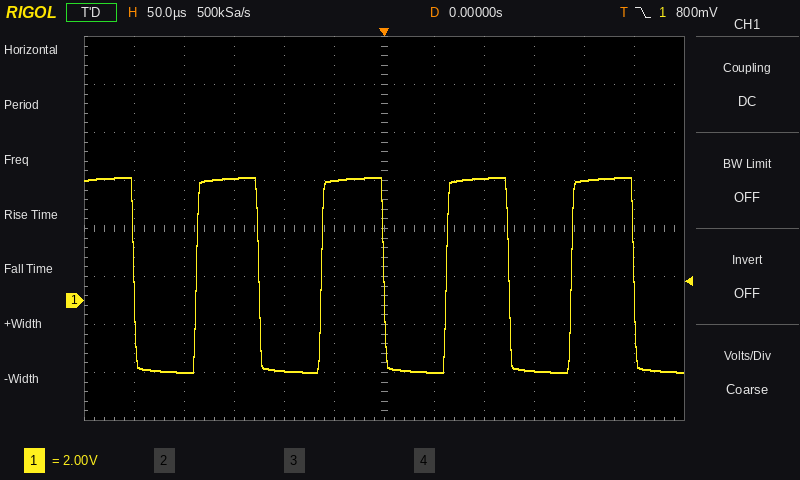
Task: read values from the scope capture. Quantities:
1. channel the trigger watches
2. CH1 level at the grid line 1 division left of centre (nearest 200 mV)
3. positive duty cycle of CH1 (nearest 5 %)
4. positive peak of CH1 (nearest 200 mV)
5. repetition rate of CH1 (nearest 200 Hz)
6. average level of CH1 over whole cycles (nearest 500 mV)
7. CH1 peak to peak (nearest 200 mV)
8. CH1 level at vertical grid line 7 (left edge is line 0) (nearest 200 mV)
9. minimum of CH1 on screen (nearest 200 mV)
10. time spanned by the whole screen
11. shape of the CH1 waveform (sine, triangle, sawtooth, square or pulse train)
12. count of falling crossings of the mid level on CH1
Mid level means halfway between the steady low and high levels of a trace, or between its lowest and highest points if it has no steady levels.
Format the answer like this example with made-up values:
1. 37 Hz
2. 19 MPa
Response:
1. CH1
2. 5.0 V
3. 50 %
4. 5.2 V
5. 8.0 kHz
6. 1.0 V
7. 8.2 V
8. -3.0 V
9. -3.0 V
10. 600 µs
11. square
12. 5
